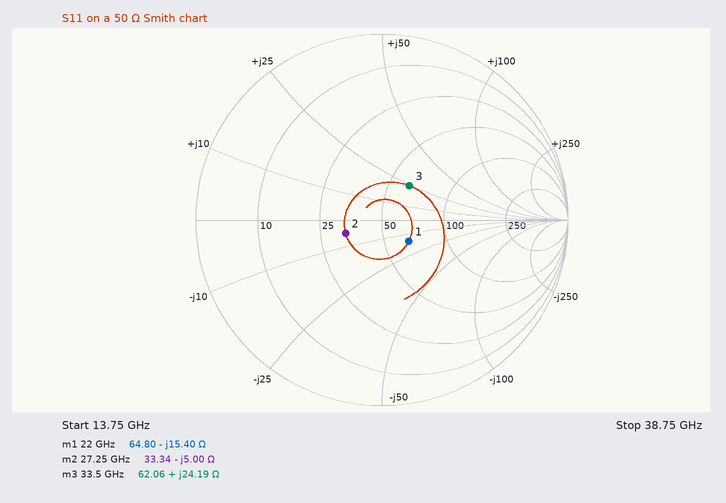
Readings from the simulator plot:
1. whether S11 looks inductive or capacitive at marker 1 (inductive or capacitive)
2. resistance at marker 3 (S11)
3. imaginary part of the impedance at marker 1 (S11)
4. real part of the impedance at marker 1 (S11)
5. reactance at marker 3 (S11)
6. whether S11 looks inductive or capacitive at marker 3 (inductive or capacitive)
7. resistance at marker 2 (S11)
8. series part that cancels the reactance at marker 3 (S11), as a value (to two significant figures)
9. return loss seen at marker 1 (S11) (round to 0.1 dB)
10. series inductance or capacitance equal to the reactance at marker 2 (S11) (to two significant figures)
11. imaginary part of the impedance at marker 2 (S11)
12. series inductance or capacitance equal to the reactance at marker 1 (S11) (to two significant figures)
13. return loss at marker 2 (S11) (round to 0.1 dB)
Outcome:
capacitive
62.06 Ω
-15.40 Ω
64.80 Ω
+24.19 Ω
inductive
33.34 Ω
200 fF
14.7 dB
1.2 pF
-5.00 Ω
470 fF
13.6 dB
